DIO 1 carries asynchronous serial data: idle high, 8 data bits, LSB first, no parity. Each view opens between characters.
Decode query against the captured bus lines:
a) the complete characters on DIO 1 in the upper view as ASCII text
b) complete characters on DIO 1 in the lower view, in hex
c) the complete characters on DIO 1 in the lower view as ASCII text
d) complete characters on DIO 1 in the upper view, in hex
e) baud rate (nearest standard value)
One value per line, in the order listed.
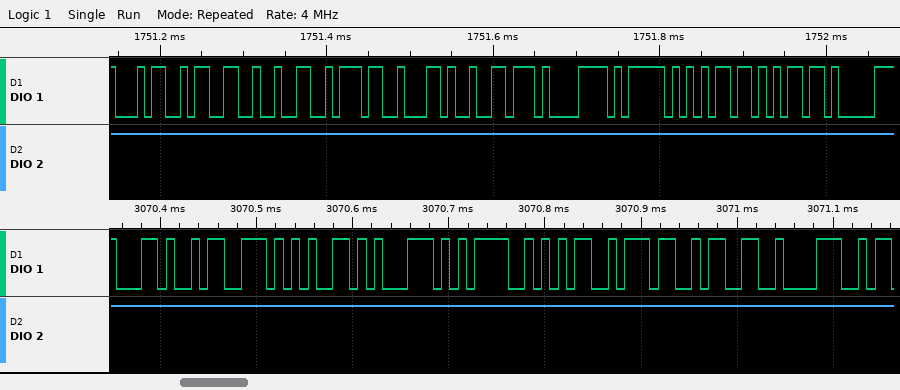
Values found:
"4327,vx_mm"
2C, 73, 65, 71, 3D, 35, 37, 33, 38
",seq=5738"
34, 33, 32, 37, 2C, 76, 78, 5F, 6D, 6D
115200 baud
